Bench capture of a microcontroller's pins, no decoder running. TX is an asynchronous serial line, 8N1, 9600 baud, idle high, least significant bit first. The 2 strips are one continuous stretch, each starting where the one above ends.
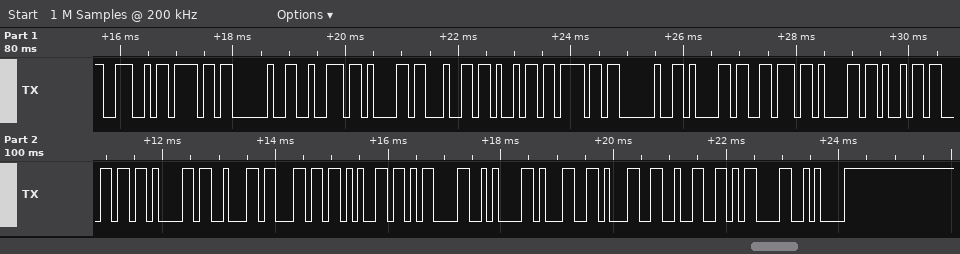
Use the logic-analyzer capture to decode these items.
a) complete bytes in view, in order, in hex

0x4E 0x6F 0x20 0x72 0x61 0x64 0x69 0x6F 0x20 0x61 0x76 0x61 0x69 0x6C 0x61 0x62 0x6C 0x65 0x0D 0x0A 0x31 0x31 0x32 0x0D 0x0A
